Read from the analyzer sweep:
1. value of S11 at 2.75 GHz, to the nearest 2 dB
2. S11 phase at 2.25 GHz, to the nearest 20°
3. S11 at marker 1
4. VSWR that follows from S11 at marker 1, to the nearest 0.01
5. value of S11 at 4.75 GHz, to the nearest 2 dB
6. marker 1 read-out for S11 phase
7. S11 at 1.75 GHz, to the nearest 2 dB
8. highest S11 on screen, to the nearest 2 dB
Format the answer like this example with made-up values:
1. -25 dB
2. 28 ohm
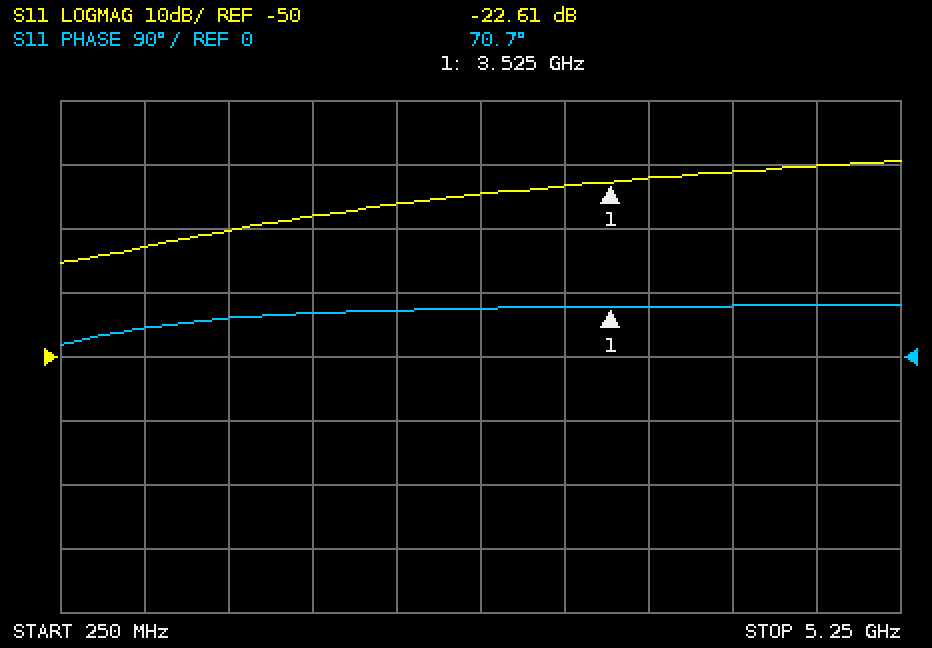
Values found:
1. -24 dB
2. 60°
3. -22.61 dB
4. 1.16
5. -20 dB
6. 70.7°
7. -28 dB
8. -20 dB
